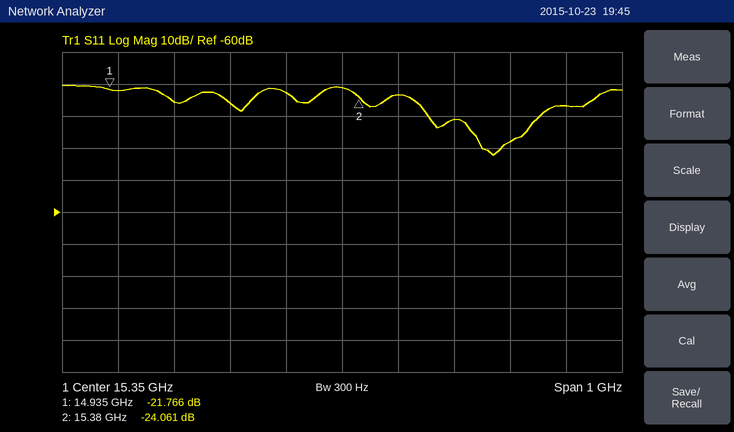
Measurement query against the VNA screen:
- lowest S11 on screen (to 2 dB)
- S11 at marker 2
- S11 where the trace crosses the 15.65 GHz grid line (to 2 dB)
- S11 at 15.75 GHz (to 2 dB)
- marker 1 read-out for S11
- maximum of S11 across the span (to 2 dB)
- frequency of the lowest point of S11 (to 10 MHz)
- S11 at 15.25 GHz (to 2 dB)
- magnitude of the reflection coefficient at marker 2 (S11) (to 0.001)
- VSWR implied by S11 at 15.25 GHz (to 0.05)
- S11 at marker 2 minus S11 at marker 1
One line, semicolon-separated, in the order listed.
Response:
-42 dB; -24.061 dB; -38 dB; -26 dB; -21.766 dB; -20 dB; 15.62 GHz; -22 dB; 0.063; 1.15; -2.295 dB
